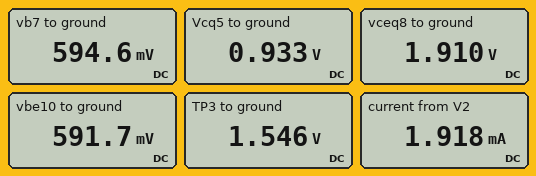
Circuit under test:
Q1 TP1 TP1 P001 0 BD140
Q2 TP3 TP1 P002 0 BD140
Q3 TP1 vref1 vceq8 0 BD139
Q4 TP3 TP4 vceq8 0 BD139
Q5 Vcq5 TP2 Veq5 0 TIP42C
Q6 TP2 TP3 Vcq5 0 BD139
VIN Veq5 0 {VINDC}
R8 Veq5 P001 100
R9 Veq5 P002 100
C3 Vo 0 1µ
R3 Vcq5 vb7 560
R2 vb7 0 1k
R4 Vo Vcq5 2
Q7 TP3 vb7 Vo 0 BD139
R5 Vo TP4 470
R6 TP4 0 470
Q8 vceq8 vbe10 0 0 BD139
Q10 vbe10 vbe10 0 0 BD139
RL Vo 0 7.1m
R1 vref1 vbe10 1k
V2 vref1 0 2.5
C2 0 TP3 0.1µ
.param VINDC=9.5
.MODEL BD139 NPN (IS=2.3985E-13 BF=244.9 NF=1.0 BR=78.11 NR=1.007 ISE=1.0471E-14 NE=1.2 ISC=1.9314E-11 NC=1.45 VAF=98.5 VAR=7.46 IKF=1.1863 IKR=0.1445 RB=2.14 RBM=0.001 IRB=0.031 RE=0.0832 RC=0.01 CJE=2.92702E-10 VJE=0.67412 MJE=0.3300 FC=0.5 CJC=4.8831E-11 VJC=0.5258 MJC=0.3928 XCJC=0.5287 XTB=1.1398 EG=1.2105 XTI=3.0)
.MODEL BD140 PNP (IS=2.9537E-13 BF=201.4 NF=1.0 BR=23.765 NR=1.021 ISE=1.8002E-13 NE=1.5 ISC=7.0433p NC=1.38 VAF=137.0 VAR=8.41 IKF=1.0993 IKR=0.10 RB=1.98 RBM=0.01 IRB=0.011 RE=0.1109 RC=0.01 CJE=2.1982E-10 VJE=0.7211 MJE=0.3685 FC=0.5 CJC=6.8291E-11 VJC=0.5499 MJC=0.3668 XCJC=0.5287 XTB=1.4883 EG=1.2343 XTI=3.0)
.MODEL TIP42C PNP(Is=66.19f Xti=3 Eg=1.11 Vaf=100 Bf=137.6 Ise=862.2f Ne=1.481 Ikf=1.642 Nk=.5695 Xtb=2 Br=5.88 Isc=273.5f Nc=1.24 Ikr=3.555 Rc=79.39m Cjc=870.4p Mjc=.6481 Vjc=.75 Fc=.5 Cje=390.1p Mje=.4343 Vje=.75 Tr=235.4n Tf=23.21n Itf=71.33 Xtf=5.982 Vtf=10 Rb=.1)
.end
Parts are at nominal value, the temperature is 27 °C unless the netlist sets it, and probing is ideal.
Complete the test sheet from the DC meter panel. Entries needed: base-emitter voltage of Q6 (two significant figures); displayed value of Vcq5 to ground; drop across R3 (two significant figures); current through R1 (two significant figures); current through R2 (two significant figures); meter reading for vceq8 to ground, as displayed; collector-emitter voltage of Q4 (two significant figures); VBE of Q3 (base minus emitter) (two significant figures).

610 mV
0.933 V
340 mV
1.9 mA
590 µA
1.910 V
-360 mV
590 mV
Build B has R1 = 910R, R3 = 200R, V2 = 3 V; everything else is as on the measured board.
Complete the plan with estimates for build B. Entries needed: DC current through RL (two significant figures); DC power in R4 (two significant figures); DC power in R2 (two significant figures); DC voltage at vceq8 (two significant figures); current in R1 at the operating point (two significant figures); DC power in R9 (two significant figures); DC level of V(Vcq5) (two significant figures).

360 mA
260 mW
360 µW
2.4 V
2.6 mA
700 µW
730 mV
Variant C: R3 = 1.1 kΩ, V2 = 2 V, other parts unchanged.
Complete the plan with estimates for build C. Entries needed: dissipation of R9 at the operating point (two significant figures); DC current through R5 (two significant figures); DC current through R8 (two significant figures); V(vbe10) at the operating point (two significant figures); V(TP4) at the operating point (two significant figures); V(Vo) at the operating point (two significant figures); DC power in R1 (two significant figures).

200 µW
4.7 µA
1.4 mA
580 mV
2.2 mV
4.4 mV
2.0 mW
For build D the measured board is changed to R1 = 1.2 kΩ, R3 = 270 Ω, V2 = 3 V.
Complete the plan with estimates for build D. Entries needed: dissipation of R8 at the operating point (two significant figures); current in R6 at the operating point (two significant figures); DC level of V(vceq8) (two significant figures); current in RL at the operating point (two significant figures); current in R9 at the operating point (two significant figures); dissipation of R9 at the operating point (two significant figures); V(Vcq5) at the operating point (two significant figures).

400 µW
2.9 µA
2.4 V
380 mA
2.0 mA
410 µW
760 mV
